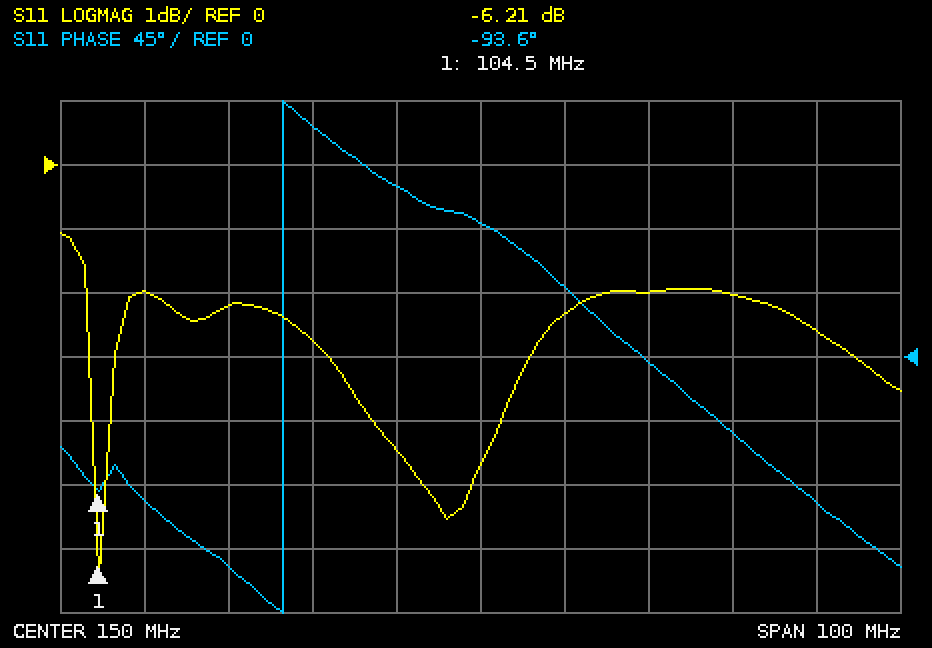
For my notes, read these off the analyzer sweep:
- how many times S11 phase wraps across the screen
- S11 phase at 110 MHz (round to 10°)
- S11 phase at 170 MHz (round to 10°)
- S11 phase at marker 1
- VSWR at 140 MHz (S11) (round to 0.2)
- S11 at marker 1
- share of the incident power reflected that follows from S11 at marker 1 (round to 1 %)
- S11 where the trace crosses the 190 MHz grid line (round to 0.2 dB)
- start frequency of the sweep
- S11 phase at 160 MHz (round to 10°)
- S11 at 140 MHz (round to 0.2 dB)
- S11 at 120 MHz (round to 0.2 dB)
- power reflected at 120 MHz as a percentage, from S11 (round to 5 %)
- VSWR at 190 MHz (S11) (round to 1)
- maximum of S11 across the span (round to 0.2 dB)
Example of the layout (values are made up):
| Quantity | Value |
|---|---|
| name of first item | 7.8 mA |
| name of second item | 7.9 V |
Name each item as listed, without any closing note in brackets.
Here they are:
| Quantity | Value |
|---|---|
| how many times S11 phase wraps across the screen | 1 |
| S11 phase at 110 MHz | -100° |
| S11 phase at 170 MHz | 0° |
| S11 phase at marker 1 | -93.6° |
| VSWR at 140 MHz (S11) | 4.0 |
| S11 at marker 1 | -6.21 dB |
| share of the incident power reflected that follows from S11 at marker 1 | 24 % |
| S11 where the trace crosses the 190 MHz grid line | -2.6 dB |
| start frequency of the sweep | 100 MHz |
| S11 phase at 160 MHz | 50° |
| S11 at 140 MHz | -4.4 dB |
| S11 at 120 MHz | -2.2 dB |
| power reflected at 120 MHz as a percentage, from S11 | 60 % |
| VSWR at 190 MHz (S11) | 7 |
| maximum of S11 across the span | -1.0 dB |
